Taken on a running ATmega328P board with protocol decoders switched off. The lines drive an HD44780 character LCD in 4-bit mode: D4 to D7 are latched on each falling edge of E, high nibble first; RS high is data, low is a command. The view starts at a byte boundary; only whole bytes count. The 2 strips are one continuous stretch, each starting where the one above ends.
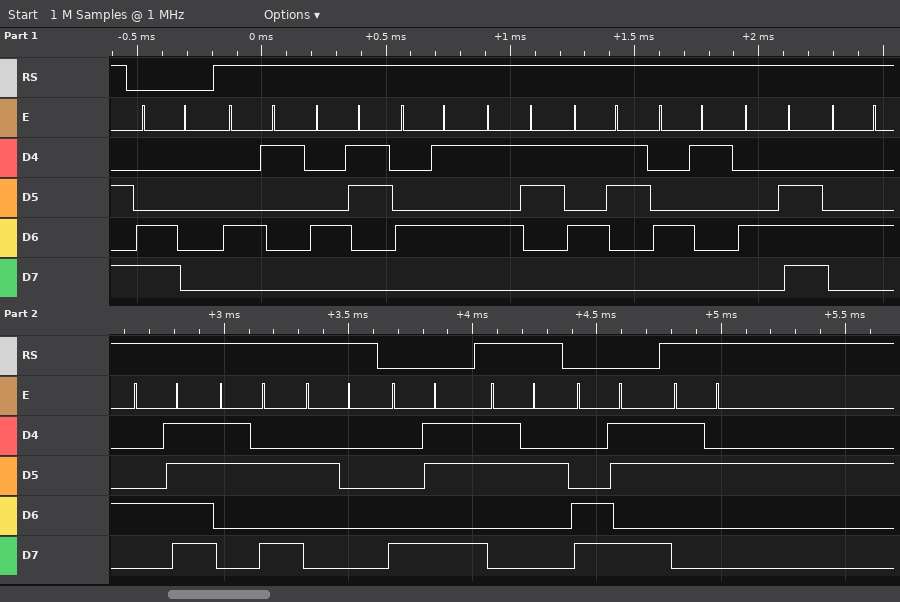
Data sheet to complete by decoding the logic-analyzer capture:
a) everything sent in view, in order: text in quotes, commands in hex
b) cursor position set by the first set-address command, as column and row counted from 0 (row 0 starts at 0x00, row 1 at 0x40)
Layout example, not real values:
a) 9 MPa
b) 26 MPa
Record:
a) 0xC0 "ACESSANDO: " 0x8B "2" 0xCB "2"
b) column 0, row 1
